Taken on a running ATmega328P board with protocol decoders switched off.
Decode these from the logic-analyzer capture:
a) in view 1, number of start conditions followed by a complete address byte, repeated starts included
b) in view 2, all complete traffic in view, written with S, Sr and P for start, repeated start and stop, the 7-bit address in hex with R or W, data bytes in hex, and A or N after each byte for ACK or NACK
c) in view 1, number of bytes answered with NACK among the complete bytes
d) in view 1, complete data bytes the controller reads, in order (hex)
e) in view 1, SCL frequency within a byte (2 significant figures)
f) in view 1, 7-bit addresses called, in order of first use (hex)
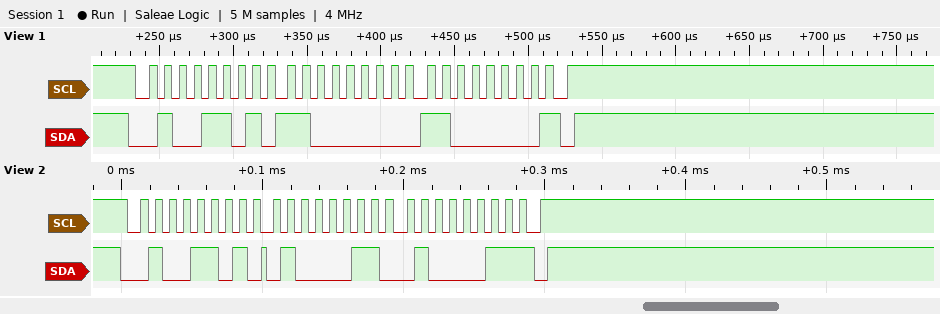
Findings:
1
S 26R A 43 A 43 N P
1
C0 C0
100 kHz
0x26
